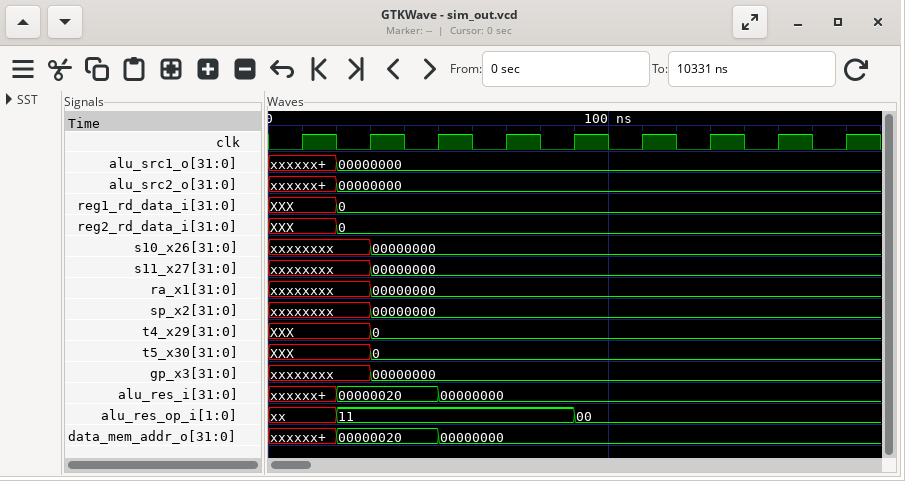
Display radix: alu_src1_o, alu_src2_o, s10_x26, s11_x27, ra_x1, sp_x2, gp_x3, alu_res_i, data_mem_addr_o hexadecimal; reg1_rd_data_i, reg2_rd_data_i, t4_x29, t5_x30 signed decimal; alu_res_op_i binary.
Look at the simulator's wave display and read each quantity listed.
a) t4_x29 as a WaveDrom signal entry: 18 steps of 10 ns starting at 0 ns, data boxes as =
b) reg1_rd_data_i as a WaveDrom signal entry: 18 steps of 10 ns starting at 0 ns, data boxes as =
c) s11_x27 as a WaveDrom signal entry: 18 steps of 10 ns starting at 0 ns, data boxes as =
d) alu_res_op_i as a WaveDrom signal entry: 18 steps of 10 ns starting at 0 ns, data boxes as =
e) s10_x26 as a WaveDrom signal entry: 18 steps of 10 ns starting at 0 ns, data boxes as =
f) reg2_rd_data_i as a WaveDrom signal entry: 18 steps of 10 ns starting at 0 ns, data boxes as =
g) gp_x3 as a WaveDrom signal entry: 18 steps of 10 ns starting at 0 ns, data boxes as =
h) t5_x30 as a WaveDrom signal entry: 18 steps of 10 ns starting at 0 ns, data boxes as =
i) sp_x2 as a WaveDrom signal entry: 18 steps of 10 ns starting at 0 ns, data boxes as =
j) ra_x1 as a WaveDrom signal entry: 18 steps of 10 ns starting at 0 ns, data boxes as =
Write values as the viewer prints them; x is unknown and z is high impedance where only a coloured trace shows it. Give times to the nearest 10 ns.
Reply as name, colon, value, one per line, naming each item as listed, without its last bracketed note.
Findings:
t4_x29 as a WaveDrom signal entry: 18 steps of 10 ns starting at 0 ns, data boxes as =: {name: 't4_x29', wave: 'x..=..............', data: '0'}
reg1_rd_data_i as a WaveDrom signal entry: 18 steps of 10 ns starting at 0 ns, data boxes as =: {name: 'reg1_rd_data_i', wave: 'x.=...............', data: '0'}
s11_x27 as a WaveDrom signal entry: 18 steps of 10 ns starting at 0 ns, data boxes as =: {name: 's11_x27', wave: 'x..=..............', data: '00000000'}
alu_res_op_i as a WaveDrom signal entry: 18 steps of 10 ns starting at 0 ns, data boxes as =: {name: 'alu_res_op_i', wave: 'x.=......=........', data: '11 00'}
s10_x26 as a WaveDrom signal entry: 18 steps of 10 ns starting at 0 ns, data boxes as =: {name: 's10_x26', wave: 'x..=..............', data: '00000000'}
reg2_rd_data_i as a WaveDrom signal entry: 18 steps of 10 ns starting at 0 ns, data boxes as =: {name: 'reg2_rd_data_i', wave: 'x.=...............', data: '0'}
gp_x3 as a WaveDrom signal entry: 18 steps of 10 ns starting at 0 ns, data boxes as =: {name: 'gp_x3', wave: 'x..=..............', data: '00000000'}
t5_x30 as a WaveDrom signal entry: 18 steps of 10 ns starting at 0 ns, data boxes as =: {name: 't5_x30', wave: 'x..=..............', data: '0'}
sp_x2 as a WaveDrom signal entry: 18 steps of 10 ns starting at 0 ns, data boxes as =: {name: 'sp_x2', wave: 'x..=..............', data: '00000000'}
ra_x1 as a WaveDrom signal entry: 18 steps of 10 ns starting at 0 ns, data boxes as =: {name: 'ra_x1', wave: 'x..=..............', data: '00000000'}
